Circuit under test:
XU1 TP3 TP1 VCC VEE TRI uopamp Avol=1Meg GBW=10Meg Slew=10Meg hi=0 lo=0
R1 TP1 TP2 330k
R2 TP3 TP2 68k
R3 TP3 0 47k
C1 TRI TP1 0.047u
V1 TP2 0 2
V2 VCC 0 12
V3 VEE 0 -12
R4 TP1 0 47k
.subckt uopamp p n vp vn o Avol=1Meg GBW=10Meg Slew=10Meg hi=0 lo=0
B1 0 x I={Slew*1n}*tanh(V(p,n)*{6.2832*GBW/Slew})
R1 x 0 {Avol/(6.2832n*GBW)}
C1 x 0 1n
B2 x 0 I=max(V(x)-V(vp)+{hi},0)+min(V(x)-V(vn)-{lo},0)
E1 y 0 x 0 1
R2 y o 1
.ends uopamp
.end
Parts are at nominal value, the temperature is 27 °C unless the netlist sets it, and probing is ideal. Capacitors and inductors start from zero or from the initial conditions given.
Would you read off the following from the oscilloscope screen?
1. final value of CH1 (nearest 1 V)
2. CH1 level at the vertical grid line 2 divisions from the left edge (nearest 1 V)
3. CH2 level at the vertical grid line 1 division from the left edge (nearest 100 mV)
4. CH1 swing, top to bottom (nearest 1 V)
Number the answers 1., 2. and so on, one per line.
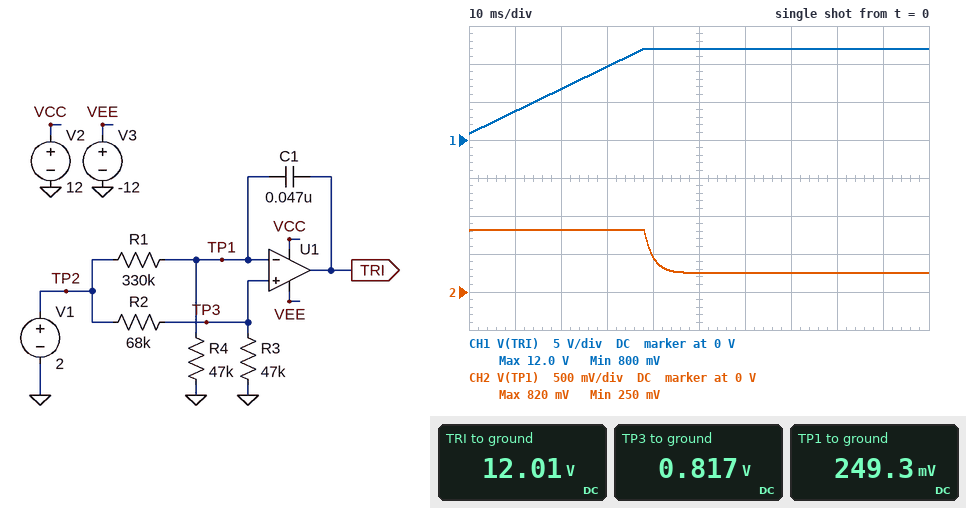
1. 12 V
2. 7 V
3. 800 mV
4. 11 V
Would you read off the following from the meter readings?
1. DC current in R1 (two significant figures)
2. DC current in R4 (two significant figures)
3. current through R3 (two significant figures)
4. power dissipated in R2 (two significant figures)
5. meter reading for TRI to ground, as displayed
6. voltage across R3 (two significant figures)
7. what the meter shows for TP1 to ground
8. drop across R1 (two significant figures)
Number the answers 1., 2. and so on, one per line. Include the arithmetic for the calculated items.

1. (2 V - 249.3 mV) / 330 kΩ = 5.3 µA
2. (249.3 mV) / 47 kΩ = 5.3 µA
3. (817 mV) / 47 kΩ = 17 µA
4. (2 V - 817 mV)^2 / 68 kΩ = 21 µW
5. 12.01 V
6. 817 mV = 820 mV
7. 249.3 mV
8. 2 V - 249.3 mV = 1.8 V
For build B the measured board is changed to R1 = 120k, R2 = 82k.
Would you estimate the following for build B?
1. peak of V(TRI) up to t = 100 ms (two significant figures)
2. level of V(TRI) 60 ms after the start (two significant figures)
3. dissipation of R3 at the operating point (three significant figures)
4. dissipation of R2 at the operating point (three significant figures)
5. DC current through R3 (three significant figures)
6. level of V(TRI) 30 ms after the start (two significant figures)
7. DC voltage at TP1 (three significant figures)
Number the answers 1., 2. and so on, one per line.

1. 11 V
2. 7.0 V
3. 11.3 µW
4. 19.7 µW
5. 15.5 µA
6. 3.9 V
7. 563 mV
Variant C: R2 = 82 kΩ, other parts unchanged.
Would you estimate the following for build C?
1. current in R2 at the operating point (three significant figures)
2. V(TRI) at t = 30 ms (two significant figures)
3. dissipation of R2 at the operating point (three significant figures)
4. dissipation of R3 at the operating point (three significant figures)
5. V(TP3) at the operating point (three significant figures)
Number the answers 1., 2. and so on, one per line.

1. 15.5 µA
2. 8.2 V
3. 19.7 µW
4. 11.3 µW
5. 729 mV
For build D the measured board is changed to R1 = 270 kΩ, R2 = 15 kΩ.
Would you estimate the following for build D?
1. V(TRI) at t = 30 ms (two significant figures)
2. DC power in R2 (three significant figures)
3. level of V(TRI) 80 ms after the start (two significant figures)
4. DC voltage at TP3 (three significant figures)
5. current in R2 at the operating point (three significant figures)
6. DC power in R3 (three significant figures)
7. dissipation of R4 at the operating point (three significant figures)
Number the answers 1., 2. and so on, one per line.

1. 12 V
2. 15.6 µW
3. 12 V
4. 1.52 V
5. 32.3 µA
6. 48.9 µW
7. 1.87 µW
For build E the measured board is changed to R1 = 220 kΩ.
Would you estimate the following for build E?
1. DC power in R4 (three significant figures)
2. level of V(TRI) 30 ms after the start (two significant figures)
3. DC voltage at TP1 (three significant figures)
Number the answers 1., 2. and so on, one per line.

1. 2.64 µW
2. 8.5 V
3. 352 mV
